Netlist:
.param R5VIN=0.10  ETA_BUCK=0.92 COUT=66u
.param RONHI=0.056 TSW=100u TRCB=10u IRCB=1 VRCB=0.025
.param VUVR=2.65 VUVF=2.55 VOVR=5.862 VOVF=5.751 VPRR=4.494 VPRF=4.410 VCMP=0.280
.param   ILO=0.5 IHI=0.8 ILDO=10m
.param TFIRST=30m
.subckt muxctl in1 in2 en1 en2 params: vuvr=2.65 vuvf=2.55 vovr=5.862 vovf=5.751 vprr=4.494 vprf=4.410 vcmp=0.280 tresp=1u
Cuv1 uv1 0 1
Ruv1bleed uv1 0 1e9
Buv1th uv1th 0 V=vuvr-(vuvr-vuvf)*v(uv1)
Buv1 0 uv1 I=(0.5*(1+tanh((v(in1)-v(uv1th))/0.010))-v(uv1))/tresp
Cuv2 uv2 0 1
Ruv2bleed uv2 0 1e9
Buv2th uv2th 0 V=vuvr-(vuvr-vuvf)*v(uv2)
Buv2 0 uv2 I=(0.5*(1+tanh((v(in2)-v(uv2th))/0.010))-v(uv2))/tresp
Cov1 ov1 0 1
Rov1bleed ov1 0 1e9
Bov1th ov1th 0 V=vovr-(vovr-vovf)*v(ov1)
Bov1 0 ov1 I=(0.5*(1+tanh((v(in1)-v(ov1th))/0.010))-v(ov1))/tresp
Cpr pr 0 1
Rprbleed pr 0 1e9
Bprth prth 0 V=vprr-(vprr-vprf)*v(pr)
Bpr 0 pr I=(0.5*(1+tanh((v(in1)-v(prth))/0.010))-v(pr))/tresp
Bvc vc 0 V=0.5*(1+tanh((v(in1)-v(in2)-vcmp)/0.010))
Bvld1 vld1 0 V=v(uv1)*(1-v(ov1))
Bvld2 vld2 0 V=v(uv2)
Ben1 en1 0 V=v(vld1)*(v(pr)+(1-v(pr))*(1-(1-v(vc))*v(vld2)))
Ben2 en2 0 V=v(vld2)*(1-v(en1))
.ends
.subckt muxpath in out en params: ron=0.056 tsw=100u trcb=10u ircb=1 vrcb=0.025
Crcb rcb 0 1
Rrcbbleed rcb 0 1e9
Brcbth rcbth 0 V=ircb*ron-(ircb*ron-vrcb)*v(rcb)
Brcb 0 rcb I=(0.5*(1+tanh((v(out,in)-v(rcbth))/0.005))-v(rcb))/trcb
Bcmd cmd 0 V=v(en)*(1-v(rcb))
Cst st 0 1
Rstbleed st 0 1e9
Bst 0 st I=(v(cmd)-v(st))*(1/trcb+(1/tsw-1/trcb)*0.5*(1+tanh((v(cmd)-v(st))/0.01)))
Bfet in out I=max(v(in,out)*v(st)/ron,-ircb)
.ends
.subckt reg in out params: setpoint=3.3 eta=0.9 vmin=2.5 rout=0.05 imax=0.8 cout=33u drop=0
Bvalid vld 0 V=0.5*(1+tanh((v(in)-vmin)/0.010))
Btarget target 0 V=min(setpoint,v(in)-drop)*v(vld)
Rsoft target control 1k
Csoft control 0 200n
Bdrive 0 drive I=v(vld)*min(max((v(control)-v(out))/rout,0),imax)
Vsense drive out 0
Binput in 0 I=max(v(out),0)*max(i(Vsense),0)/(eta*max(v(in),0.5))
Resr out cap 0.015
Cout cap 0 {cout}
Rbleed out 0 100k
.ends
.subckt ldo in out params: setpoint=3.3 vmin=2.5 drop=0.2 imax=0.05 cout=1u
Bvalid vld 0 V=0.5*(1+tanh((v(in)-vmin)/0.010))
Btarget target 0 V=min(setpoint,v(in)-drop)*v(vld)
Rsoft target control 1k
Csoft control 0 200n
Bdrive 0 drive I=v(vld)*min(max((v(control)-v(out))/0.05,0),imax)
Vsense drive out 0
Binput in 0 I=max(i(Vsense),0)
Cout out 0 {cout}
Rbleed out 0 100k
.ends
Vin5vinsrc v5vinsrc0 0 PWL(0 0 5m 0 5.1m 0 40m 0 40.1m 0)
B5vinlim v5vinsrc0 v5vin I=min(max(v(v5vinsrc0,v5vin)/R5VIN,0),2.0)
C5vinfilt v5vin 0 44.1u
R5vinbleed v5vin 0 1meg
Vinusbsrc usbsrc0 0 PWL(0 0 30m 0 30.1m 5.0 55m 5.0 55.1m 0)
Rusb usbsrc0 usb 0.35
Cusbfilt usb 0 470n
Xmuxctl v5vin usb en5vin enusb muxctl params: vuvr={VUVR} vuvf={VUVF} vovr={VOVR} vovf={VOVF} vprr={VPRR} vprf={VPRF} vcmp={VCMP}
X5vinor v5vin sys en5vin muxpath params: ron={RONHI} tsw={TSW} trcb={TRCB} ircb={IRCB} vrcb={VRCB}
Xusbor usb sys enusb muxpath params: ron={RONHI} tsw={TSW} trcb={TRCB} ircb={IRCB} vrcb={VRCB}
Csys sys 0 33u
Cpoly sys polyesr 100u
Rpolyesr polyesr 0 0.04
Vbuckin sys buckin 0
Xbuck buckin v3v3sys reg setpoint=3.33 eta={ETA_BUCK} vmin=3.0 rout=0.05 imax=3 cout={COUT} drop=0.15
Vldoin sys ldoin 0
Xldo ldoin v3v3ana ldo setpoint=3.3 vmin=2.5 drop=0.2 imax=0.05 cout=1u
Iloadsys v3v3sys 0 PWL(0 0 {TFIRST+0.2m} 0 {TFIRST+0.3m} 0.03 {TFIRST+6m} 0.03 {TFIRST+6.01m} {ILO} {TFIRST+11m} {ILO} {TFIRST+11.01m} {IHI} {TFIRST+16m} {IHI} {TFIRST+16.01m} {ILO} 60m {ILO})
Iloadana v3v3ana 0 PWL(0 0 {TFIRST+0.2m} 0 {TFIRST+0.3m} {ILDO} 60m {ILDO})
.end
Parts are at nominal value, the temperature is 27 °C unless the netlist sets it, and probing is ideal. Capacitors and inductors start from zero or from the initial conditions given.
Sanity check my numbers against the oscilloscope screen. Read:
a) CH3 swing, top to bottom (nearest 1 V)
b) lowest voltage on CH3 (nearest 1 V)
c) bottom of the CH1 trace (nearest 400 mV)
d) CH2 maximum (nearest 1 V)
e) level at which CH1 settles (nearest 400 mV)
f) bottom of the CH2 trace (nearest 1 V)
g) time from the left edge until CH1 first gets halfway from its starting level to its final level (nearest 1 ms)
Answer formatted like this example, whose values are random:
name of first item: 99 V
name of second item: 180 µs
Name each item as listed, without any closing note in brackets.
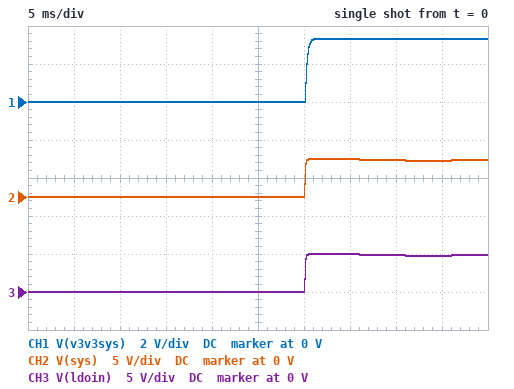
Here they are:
CH3 swing, top to bottom: 5 V
lowest voltage on CH3: 0 V
bottom of the CH1 trace: 0 V
CH2 maximum: 5 V
level at which CH1 settles: 3.2 V
bottom of the CH2 trace: 0 V
time from the left edge until CH1 first gets halfway from its starting level to its final level: 30 ms
